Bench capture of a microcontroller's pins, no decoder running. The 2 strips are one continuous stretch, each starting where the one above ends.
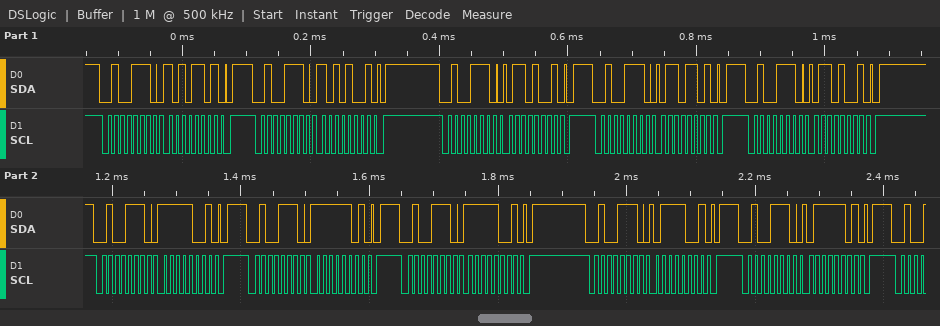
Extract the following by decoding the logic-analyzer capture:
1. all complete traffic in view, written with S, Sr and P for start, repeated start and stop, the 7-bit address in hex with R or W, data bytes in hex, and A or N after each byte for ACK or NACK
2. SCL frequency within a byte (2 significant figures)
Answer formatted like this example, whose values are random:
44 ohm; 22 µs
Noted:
S 27W A AD A P S 27W A A9 A P S 27W A 69 A P S 27W A 6D A P S 27W A 69 A P S 27W A F9 A P S 27W A FD A P S 27W A F9 A P S 27W A 79 A P S 27W A 7D A P; 100 kHz
